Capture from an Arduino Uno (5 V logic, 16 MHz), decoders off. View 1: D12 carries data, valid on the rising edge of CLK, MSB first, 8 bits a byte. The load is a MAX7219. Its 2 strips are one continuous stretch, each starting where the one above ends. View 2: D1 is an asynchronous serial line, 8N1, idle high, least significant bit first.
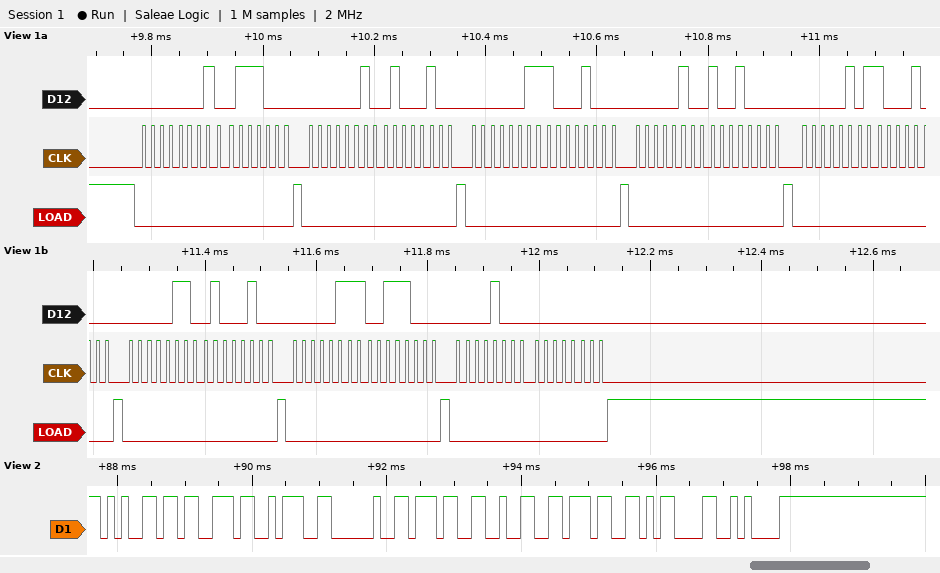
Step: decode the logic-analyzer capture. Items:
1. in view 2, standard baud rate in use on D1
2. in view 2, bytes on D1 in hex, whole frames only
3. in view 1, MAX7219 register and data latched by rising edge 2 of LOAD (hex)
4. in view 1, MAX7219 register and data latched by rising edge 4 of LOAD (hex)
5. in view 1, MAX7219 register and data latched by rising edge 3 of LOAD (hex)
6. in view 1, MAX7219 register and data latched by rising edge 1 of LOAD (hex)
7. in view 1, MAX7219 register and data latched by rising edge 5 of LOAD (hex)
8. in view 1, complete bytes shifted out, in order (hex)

9600 baud
65 73 3A 20 37 32 37 0D 0A
register 0x2, data 0x44
register 0x4, data 0x90
register 0x3, data 0x88
register 0x1, data 0x38
register 0x5, data 0x88
0x01 0x38 0x02 0x44 0x03 0x88 0x04 0x90 0x05 0x88 0x06 0x44 0x07 0x38 0x08 0x00
